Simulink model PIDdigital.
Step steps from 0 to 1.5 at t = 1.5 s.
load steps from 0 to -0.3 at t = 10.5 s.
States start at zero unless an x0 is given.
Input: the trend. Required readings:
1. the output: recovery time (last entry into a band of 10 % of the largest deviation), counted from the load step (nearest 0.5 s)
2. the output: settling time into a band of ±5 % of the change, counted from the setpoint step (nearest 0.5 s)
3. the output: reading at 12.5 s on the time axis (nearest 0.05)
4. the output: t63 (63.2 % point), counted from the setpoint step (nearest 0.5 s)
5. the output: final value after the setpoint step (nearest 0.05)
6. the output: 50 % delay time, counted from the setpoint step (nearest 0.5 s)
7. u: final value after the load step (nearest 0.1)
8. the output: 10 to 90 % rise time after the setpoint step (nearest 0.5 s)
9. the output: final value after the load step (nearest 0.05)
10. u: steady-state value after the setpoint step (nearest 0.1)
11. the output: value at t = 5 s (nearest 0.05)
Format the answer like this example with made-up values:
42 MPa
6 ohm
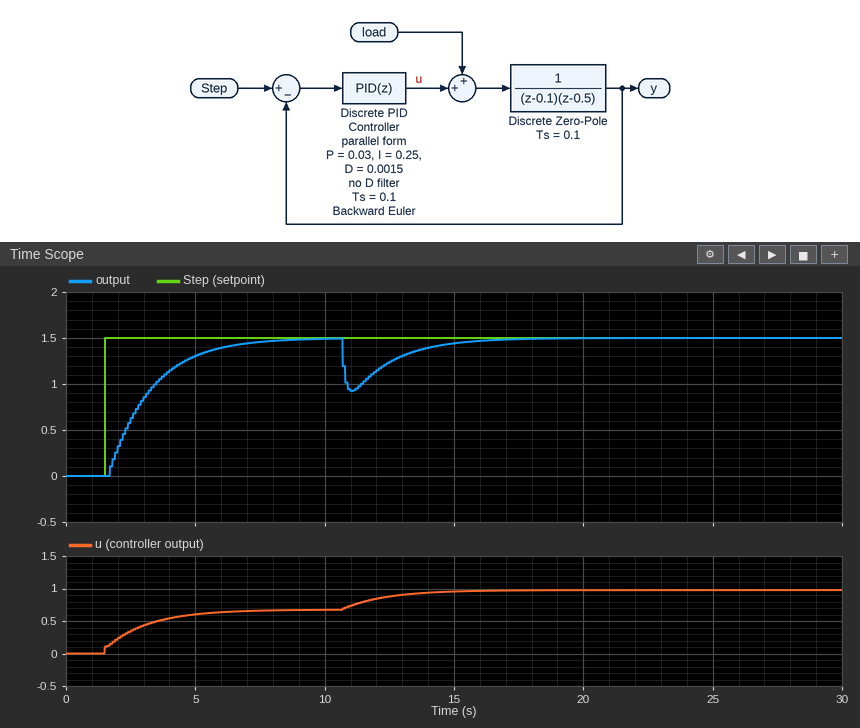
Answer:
4.5 s
5.0 s
1.25
2.0 s
1.50
1.5 s
1.0
3.5 s
1.50
0.7
1.30
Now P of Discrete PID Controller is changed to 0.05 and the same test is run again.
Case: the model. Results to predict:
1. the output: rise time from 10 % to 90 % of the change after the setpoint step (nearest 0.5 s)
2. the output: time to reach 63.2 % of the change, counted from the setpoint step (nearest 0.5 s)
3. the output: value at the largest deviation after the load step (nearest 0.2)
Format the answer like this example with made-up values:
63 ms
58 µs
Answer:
4.0 s
2.0 s
1.0
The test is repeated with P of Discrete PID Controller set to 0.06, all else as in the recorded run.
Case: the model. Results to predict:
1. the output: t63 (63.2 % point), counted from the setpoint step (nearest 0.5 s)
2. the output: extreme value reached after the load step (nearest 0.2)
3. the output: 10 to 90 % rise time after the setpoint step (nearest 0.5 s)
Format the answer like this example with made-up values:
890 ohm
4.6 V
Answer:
2.0 s
1.0
4.0 s
